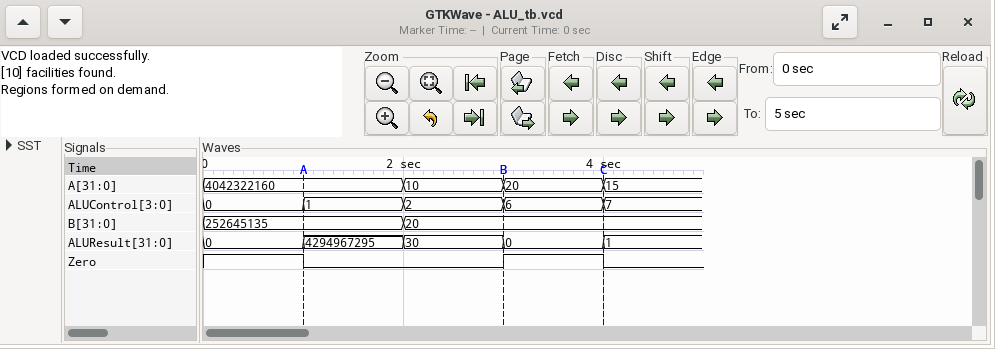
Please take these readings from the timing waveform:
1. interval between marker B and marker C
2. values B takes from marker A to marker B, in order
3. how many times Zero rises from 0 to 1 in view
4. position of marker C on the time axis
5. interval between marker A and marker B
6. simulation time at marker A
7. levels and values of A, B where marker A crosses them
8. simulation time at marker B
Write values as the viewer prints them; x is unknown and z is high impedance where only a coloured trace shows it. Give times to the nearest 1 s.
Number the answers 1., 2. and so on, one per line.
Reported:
1. 1 s
2. 252645135, 20
3. 1
4. 4 s
5. 2 s
6. 1 s
7. A=4042322160, B=252645135
8. 3 s
